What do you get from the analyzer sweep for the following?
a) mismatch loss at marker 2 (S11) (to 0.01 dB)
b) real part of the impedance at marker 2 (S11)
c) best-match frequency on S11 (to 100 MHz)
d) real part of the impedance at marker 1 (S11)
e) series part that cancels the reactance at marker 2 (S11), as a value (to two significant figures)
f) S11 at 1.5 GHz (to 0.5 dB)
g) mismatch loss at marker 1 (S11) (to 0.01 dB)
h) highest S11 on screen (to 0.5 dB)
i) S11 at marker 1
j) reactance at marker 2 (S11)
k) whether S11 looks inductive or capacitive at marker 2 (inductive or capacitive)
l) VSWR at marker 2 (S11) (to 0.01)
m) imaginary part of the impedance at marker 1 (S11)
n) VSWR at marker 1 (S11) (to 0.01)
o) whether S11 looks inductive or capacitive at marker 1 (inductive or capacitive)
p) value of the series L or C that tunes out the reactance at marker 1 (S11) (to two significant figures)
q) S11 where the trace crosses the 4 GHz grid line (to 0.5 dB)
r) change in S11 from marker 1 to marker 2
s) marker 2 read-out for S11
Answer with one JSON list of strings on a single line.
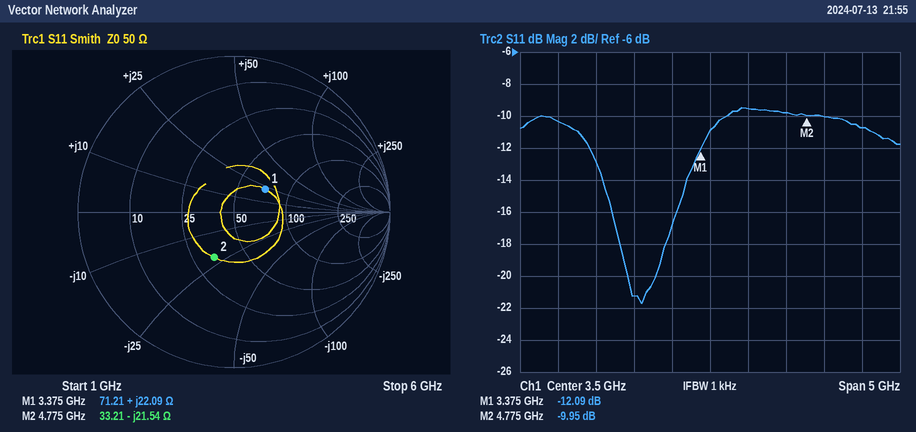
["0.46 dB", "33.21 Ω", "2.6 GHz", "71.21 Ω", "720 pH", "-10.5 dB", "0.28 dB", "-9.5 dB", "-12.09 dB", "-21.54 Ω", "capacitive", "1.93", "+22.09 Ω", "1.66", "inductive", "2.1 pF", "-9.5 dB", "2.14 dB", "-9.95 dB"]
